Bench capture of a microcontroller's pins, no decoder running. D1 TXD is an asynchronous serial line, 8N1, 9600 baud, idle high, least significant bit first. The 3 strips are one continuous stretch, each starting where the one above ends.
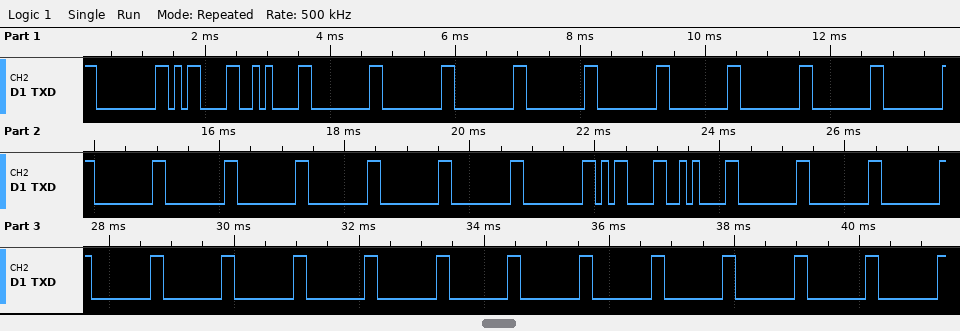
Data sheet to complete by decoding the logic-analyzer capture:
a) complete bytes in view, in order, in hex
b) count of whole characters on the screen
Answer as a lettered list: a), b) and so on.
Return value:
a) 00 0D 0A 00 00 00 00 00 00 00 00 00 00 00 00 00 00 00 00 0D 0A 00 00 00 00 00 00 00 00 00 00 00 00 00 00 00
b) 36
